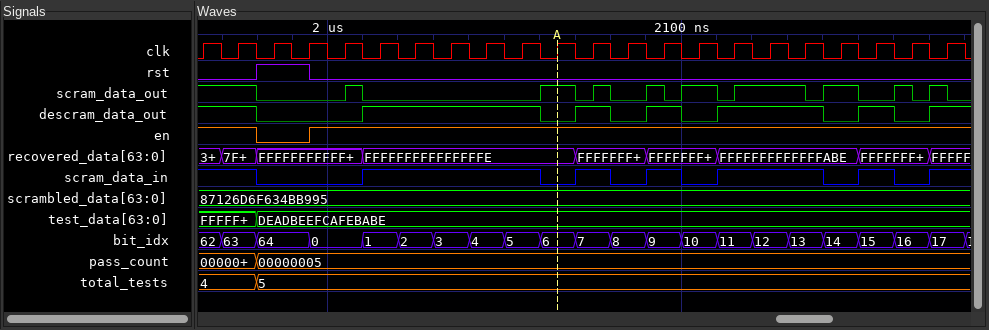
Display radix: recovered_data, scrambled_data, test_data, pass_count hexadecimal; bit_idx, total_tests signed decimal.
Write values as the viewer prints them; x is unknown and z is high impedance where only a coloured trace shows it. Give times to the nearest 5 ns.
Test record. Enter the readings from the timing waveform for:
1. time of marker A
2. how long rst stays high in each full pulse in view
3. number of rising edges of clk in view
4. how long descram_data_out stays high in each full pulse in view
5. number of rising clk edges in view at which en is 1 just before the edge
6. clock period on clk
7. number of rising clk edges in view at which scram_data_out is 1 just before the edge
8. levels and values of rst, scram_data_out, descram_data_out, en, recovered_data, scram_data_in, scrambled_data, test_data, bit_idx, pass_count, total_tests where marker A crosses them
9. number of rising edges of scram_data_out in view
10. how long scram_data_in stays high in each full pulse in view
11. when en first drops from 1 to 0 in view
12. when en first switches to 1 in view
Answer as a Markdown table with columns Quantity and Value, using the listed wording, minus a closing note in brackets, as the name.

| Quantity | Value |
|---|---|
| time of marker A | 2065 ns |
| how long rst stays high in each full pulse in view | 15 ns |
| number of rising edges of clk in view | 22 |
| how long descram_data_out stays high in each full pulse in view | 50 ns, 10 ns, 10 ns, 30 ns, 10 ns |
| number of rising clk edges in view at which en is 1 just before the edge | 20 |
| clock period on clk | 10 ns |
| number of rising clk edges in view at which scram_data_out is 1 just before the edge | 10 |
| levels and values of rst, scram_data_out, descram_data_out, en, recovered_data, scram_data_in, scrambled_data, test_data, bit_idx, pass_count, total_tests where marker A crosses them | rst=0, scram_data_out=1, descram_data_out=0, en=1, recovered_data=FFFFFFFFFFFFFFFE, scram_data_in=0, scrambled_data=87126D6F634BB995, test_data=DEADBEEFCAFEBABE, bit_idx=6, pass_count=00000005, total_tests=5 |
| number of rising edges of scram_data_out in view | 9 |
| how long scram_data_in stays high in each full pulse in view | 50 ns, 10 ns, 10 ns, 30 ns, 10 ns |
| when en first drops from 1 to 0 in view | 1980 ns |
| when en first switches to 1 in view | 1995 ns |
